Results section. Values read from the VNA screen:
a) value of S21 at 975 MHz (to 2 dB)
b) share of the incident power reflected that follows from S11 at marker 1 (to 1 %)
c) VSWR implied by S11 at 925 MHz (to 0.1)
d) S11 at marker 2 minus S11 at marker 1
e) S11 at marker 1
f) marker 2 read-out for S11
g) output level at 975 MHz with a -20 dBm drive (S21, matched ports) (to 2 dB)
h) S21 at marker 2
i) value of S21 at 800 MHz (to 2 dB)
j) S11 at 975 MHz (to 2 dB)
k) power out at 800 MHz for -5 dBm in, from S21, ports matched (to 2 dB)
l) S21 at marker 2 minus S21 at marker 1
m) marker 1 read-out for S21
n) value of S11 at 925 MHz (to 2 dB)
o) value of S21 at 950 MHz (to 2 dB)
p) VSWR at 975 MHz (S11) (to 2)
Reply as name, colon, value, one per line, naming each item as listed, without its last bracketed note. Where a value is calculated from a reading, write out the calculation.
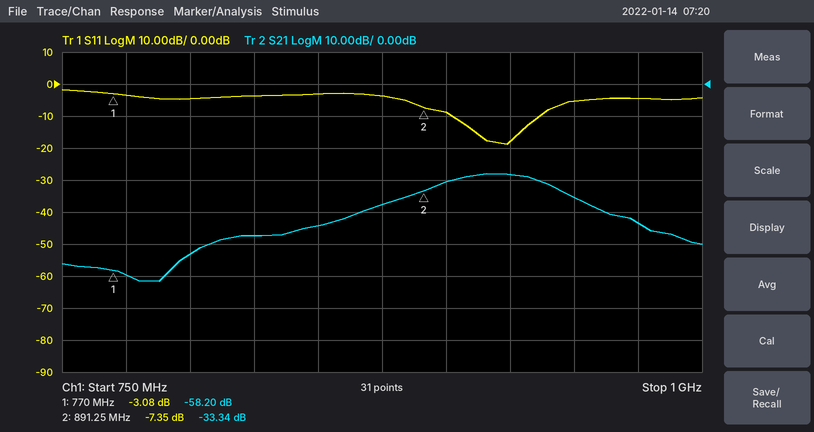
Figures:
value of S21 at 975 MHz: -44 dB
share of the incident power reflected that follows from S11 at marker 1: 10^(-3.08/10) ≈ 49 %
VSWR implied by S11 at 925 MHz: |Γ| = 10^(-18/20) = 0.1259; VSWR = (1 + 0.1259)/(1 − 0.1259) ≈ 1.3
S11 at marker 2 minus S11 at marker 1: -7.35 − (-3.08) = -4.27 dB
S11 at marker 1: -3.08 dB
marker 2 read-out for S11: -7.35 dB
output level at 975 MHz with a -20 dBm drive (S21, matched ports): -20 dBm + (-44 dB) = -64 dBm
S21 at marker 2: -33.34 dB
value of S21 at 800 MHz: -54 dB
S11 at 975 MHz: -4 dB
power out at 800 MHz for -5 dBm in, from S21, ports matched: -5 dBm + (-54 dB) = -58 dBm
S21 at marker 2 minus S21 at marker 1: -33.34 − (-58.2) = 24.86 dB
marker 1 read-out for S21: -58.20 dB
value of S11 at 925 MHz: -18 dB
value of S21 at 950 MHz: -36 dB
VSWR at 975 MHz (S11): |Γ| = 10^(-4/20) = 0.6310; VSWR = (1 + 0.6310)/(1 − 0.6310) ≈ 4
